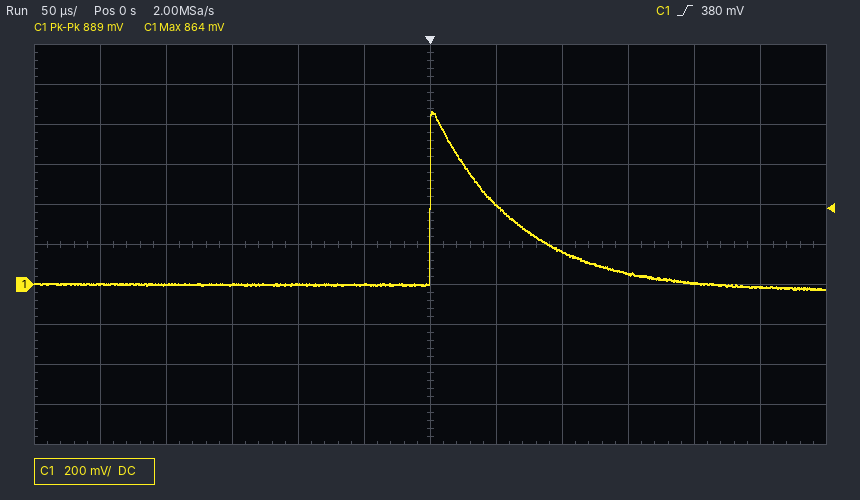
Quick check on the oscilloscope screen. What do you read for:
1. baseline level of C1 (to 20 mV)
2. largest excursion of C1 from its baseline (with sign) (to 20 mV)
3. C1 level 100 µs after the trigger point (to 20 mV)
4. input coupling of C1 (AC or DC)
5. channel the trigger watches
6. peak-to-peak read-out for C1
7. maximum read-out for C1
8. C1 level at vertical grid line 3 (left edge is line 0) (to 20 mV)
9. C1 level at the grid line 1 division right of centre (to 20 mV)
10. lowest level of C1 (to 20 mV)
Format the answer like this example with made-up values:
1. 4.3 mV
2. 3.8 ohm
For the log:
1. 0 mV
2. +860 mV
3. 160 mV
4. DC
5. C1
6. 889 mV
7. 864 mV
8. 0 mV
9. 400 mV
10. -20 mV
